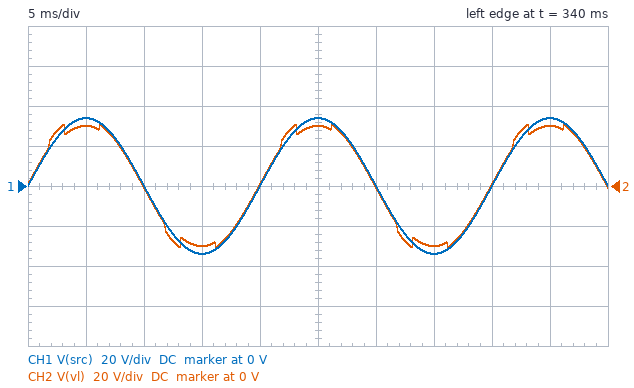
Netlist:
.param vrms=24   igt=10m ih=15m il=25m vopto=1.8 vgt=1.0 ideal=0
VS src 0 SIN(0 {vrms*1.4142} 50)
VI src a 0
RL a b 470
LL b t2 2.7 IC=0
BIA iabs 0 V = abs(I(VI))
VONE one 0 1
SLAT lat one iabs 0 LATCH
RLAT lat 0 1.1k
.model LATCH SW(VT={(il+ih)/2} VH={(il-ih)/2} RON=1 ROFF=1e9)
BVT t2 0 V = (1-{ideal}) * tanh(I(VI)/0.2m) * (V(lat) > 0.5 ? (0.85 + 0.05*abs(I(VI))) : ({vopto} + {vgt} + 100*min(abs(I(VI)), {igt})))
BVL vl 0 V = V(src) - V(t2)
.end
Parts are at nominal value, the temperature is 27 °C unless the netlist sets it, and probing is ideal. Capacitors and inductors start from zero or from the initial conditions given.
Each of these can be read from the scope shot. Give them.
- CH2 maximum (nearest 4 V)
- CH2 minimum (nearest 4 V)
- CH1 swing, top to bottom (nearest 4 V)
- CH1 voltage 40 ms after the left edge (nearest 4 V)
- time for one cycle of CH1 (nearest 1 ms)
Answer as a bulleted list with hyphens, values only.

- 32 V
- -32 V
- 68 V
- 0 V
- 20 ms
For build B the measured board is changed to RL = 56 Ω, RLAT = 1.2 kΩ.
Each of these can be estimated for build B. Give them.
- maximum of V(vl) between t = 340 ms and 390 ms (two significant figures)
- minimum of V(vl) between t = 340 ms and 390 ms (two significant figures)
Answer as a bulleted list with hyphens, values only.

- 36 V
- -36 V
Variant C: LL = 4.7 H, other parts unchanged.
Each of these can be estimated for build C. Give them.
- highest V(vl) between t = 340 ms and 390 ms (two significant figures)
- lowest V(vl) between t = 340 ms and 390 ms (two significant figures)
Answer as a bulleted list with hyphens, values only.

- 33 V
- -33 V
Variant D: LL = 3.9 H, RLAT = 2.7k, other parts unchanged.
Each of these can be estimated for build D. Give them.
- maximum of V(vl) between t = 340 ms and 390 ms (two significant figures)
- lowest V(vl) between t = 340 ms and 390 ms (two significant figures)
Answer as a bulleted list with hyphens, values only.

- 32 V
- -32 V
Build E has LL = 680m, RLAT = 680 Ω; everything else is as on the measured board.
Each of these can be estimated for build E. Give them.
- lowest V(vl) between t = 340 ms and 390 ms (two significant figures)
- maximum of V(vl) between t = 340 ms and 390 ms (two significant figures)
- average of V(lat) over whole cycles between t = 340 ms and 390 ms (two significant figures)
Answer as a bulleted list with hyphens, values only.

- -33 V
- 33 V
- 770 mV
